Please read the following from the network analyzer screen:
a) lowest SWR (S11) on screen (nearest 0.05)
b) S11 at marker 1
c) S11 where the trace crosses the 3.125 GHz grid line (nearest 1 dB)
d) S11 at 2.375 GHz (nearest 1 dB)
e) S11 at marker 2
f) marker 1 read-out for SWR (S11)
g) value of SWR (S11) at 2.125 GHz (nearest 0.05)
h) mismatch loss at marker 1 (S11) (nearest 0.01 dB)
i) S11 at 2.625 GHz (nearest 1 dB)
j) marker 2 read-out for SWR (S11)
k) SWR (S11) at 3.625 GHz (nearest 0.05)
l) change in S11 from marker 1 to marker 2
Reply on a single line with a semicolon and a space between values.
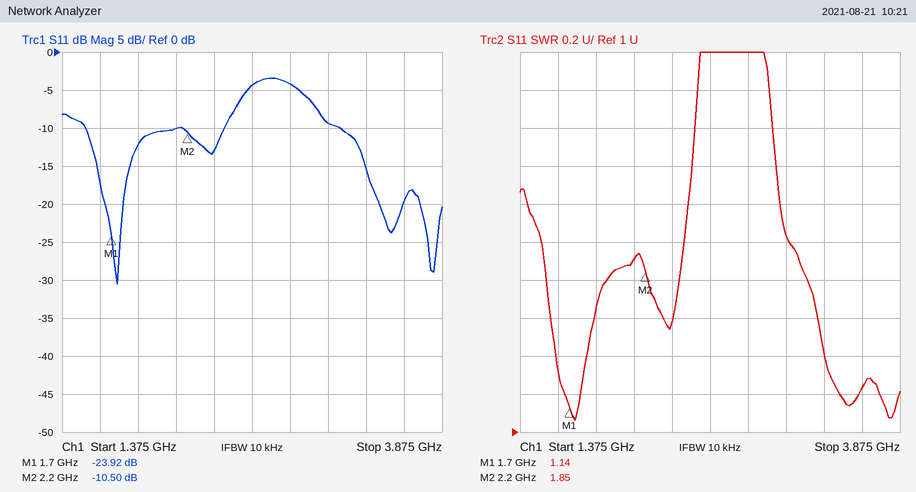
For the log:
1.05; -23.92 dB; -9 dB; -13 dB; -10.50 dB; 1.14; 1.90; 0.02 dB; -4 dB; 1.85; 1.25; 13.42 dB
